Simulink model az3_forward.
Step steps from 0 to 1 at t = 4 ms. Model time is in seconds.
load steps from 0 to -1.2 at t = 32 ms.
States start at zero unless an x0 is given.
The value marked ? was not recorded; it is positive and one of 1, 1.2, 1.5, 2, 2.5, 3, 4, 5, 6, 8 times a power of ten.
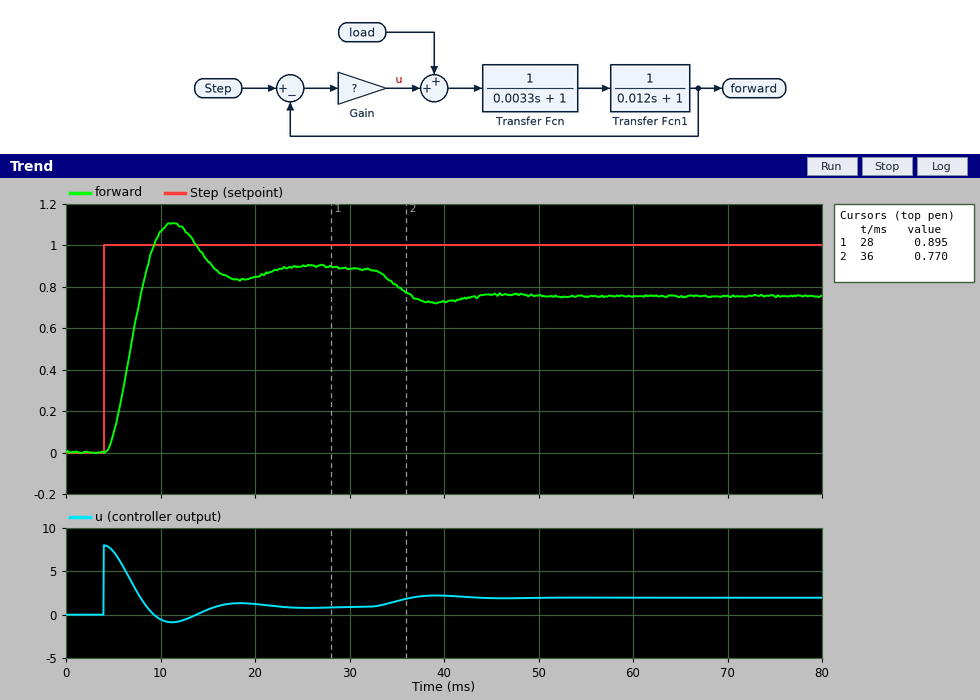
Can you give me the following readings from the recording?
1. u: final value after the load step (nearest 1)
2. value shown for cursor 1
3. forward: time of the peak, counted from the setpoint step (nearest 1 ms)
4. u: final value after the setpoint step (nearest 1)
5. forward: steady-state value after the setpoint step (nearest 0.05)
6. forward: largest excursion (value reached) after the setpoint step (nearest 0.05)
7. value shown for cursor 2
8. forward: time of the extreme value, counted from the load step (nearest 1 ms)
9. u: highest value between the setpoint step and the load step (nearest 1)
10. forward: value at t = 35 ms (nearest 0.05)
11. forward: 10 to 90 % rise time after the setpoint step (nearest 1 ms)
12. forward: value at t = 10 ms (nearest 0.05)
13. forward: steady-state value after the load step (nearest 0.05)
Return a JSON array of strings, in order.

["2", "0.895", "7 ms", "1", "0.90", "1.10", "0.770", "7 ms", "8", "0.80", "3 ms", "1.05", "0.75"]
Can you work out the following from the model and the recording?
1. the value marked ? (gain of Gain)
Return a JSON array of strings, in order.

["8"]
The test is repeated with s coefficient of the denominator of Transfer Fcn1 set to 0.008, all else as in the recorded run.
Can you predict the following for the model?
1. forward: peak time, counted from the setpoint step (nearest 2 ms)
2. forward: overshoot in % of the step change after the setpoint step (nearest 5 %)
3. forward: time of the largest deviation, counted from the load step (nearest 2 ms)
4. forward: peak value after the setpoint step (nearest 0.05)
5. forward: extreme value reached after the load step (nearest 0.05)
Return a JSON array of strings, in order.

["6 ms", "30 %", "6 ms", "1.15", "0.70"]
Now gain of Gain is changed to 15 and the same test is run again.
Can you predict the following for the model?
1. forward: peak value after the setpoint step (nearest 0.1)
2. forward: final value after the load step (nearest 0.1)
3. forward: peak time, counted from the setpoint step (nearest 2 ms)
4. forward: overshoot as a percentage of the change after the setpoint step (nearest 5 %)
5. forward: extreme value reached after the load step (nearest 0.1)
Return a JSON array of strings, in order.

["1.3", "0.9", "6 ms", "35 %", "0.8"]
